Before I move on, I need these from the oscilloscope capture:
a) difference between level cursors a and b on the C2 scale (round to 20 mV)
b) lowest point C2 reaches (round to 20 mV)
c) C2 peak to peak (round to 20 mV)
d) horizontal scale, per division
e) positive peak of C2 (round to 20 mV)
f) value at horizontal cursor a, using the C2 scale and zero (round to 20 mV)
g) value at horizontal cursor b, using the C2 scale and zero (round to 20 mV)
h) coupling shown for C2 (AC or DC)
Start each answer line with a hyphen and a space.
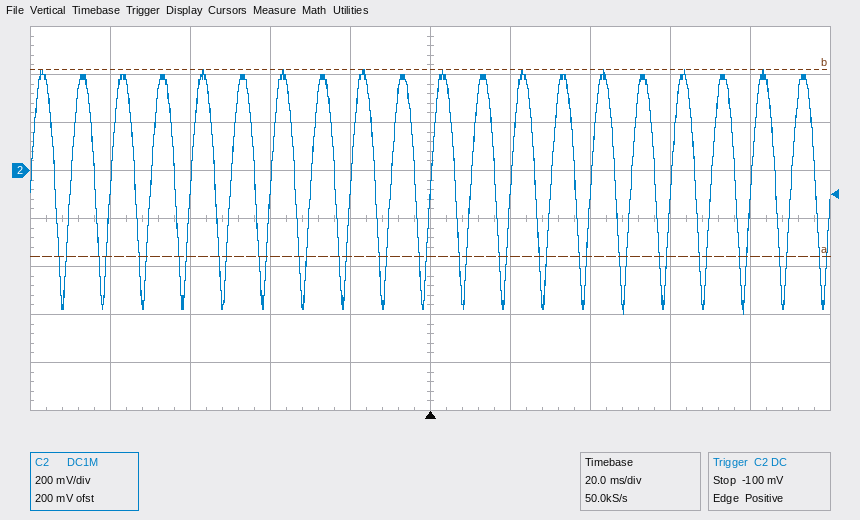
- 780 mV
- -600 mV
- 1.02 V
- 20 ms
- 420 mV
- -360 mV
- 420 mV
- DC
